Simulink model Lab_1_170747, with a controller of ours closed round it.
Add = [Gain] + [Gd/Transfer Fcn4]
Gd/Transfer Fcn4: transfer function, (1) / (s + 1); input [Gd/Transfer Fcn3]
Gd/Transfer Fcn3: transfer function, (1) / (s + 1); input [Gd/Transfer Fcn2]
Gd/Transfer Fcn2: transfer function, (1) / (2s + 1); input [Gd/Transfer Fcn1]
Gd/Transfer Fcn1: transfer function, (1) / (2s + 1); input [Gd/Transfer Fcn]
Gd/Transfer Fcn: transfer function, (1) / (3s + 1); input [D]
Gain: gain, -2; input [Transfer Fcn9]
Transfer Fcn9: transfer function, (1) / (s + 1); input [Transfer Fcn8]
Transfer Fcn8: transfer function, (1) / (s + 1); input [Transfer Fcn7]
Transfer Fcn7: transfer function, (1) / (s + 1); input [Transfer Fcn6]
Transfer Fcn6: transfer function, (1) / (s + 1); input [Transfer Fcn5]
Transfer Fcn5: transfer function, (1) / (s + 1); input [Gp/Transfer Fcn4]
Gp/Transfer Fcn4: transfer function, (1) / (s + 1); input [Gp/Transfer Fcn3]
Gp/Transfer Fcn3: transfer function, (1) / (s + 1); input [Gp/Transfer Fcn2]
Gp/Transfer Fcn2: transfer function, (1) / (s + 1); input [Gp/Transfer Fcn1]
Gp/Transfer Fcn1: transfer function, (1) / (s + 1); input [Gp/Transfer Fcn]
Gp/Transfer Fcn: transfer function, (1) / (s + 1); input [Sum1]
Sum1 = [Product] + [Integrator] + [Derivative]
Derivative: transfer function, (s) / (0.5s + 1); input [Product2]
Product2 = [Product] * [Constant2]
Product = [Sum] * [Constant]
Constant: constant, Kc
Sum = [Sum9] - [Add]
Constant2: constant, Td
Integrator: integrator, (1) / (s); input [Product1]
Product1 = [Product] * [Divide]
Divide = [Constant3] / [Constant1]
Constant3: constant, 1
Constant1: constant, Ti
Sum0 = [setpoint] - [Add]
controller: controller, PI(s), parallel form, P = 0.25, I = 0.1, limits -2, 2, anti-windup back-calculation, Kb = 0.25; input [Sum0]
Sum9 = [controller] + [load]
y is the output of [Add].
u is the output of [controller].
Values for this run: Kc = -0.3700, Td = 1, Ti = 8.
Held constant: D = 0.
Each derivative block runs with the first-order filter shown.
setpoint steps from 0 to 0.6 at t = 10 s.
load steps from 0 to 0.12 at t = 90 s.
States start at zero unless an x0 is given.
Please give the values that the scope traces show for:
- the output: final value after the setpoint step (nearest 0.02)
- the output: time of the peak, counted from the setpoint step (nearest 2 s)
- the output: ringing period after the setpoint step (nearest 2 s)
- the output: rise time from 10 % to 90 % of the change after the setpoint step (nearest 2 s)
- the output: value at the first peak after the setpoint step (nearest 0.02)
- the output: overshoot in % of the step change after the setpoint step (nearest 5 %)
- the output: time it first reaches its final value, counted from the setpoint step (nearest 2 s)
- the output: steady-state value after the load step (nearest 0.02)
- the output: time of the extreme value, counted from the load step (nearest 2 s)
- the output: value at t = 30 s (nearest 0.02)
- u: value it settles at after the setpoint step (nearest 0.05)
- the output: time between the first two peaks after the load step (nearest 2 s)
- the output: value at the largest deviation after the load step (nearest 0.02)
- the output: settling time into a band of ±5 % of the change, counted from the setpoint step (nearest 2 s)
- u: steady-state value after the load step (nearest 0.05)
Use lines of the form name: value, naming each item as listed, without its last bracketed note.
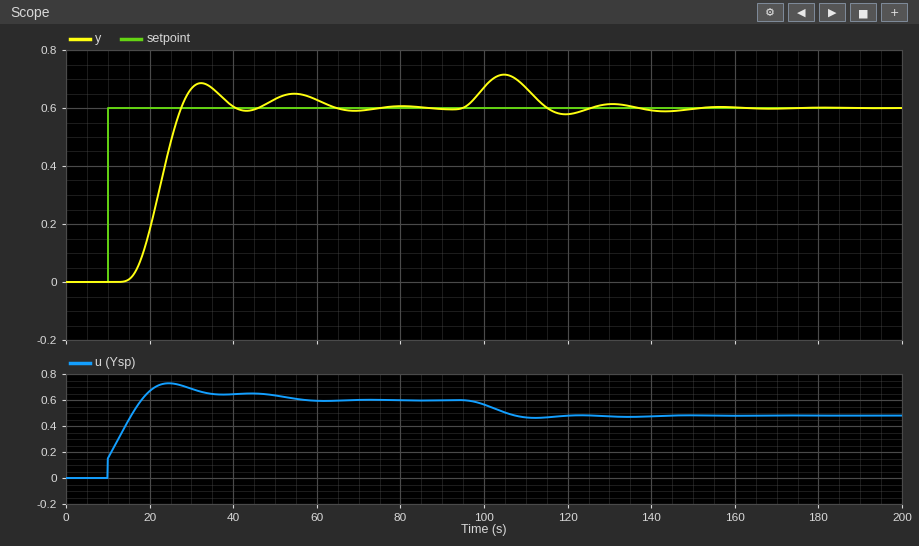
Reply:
the output: final value after the setpoint step: 0.60
the output: time of the peak, counted from the setpoint step: 22 s
the output: ringing period after the setpoint step: 22 s
the output: rise time from 10 % to 90 % of the change after the setpoint step: 8 s
the output: value at the first peak after the setpoint step: 0.68
the output: overshoot in % of the step change after the setpoint step: 15 %
the output: time it first reaches its final value, counted from the setpoint step: 18 s
the output: steady-state value after the load step: 0.60
the output: time of the extreme value, counted from the load step: 14 s
the output: value at t = 30 s: 0.66
u: value it settles at after the setpoint step: 0.60
the output: time between the first two peaks after the load step: 26 s
the output: value at the largest deviation after the load step: 0.72
the output: settling time into a band of ±5 % of the change, counted from the setpoint step: 50 s
u: steady-state value after the load step: 0.50
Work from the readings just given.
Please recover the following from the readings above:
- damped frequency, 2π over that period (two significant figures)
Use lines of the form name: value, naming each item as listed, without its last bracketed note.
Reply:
damped frequency, 2π over that period: 0.29 rad/s
